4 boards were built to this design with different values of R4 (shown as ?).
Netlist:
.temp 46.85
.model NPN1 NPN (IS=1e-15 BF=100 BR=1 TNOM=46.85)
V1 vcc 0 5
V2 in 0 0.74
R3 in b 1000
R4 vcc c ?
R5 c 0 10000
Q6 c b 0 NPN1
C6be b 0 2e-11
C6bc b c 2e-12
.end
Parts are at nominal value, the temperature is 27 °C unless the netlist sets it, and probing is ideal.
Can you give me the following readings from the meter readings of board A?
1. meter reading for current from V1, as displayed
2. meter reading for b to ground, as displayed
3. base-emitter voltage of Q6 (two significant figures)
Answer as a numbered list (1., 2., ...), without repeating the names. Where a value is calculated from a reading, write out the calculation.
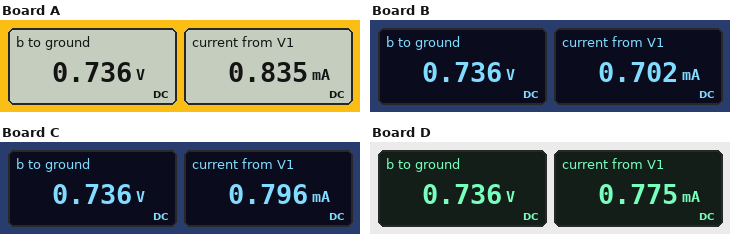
1. 0.835 mA
2. 0.736 V
3. 736 mV = 740 mV
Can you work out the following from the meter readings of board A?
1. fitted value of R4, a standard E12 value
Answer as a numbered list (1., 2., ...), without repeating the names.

1. 680 Ω
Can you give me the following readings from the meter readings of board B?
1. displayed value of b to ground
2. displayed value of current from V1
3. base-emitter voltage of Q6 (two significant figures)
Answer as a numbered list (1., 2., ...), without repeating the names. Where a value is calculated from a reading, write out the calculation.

1. 0.736 V
2. 0.702 mA
3. 736 mV = 740 mV
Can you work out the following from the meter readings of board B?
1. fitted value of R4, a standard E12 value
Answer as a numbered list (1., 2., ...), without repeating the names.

1. 2.7 kΩ
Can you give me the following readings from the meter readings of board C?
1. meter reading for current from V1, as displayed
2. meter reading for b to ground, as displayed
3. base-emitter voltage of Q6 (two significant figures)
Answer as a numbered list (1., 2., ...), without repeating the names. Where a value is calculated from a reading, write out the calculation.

1. 0.796 mA
2. 0.736 V
3. 736 mV = 740 mV
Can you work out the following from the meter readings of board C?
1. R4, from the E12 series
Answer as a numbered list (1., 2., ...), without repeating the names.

1. 1.2 kΩ
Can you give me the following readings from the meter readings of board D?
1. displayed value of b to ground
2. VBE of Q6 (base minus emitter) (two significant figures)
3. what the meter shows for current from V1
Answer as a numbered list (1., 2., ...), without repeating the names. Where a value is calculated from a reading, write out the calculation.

1. 0.736 V
2. 736 mV = 740 mV
3. 0.775 mA
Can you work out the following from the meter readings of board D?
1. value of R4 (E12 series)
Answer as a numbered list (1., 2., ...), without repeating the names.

1. 1.5 kΩ
